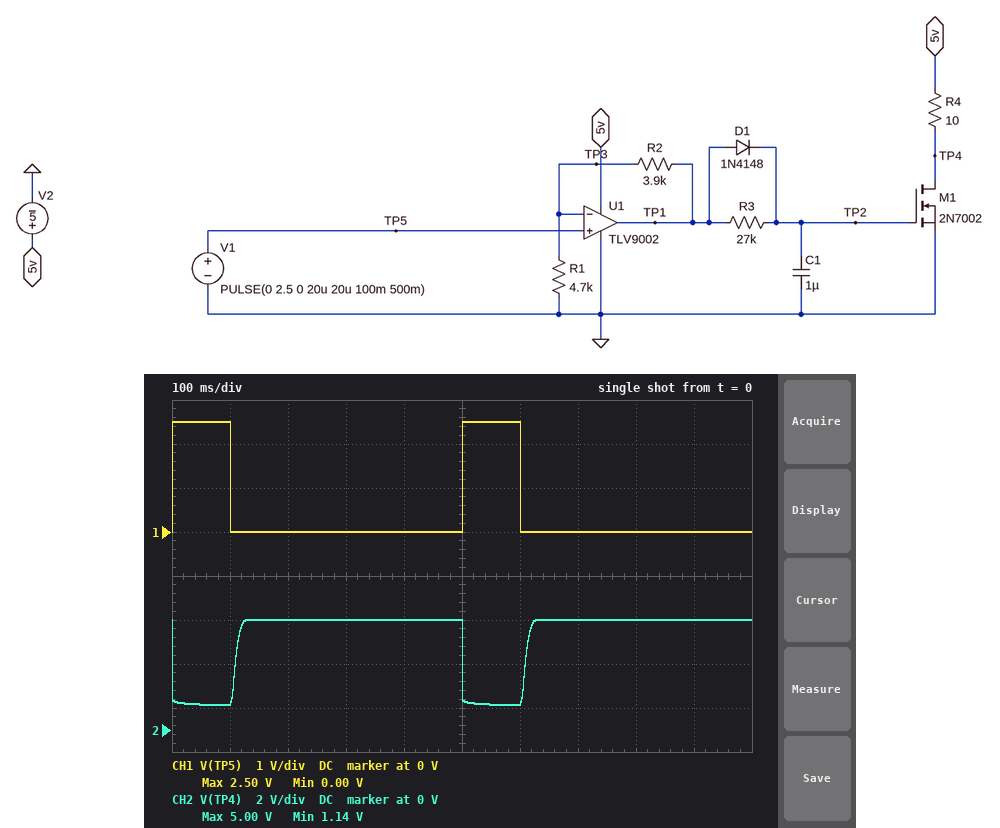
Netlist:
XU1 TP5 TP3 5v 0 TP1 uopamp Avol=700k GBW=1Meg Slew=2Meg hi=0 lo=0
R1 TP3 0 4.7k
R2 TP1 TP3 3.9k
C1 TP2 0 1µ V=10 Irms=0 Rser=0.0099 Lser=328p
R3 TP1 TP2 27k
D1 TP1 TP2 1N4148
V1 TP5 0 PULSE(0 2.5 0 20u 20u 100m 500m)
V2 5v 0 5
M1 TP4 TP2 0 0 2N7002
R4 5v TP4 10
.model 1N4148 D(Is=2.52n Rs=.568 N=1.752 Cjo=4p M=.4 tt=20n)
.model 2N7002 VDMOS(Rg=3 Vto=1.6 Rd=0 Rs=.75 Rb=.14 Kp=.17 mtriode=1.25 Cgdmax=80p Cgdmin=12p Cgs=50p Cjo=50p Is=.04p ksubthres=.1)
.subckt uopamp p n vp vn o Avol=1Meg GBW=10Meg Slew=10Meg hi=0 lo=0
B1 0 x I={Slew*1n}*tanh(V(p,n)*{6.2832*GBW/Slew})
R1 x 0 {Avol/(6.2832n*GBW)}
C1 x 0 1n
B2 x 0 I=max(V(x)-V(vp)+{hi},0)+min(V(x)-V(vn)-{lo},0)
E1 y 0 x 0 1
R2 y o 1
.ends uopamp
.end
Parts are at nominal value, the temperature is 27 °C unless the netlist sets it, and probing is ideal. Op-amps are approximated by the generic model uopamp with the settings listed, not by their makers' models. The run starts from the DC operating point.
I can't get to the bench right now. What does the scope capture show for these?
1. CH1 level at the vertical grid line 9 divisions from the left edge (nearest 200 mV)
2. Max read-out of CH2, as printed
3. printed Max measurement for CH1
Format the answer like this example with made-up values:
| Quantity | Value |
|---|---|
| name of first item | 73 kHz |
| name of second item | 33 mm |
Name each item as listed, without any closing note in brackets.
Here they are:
| Quantity | Value |
|---|---|
| CH1 level at the vertical grid line 9 divisions from the left edge | 0 V |
| Max read-out of CH2, as printed | 5.00 V |
| printed Max measurement for CH1 | 2.50 V |
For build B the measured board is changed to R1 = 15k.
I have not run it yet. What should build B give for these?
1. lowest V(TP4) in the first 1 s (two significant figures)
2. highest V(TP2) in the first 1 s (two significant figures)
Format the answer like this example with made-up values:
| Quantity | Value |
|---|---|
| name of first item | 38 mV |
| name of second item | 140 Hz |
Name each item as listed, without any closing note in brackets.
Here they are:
| Quantity | Value |
|---|---|
| lowest V(TP4) in the first 1 s | 3.3 V |
| highest V(TP2) in the first 1 s | 3.1 V |
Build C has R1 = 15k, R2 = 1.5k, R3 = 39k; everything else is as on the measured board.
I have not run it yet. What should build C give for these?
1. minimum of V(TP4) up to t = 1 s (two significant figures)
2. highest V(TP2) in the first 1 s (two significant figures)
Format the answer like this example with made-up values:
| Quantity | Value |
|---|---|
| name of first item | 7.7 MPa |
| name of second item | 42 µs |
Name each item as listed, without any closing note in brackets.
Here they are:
| Quantity | Value |
|---|---|
| minimum of V(TP4) up to t = 1 s | 4.1 V |
| highest V(TP2) in the first 1 s | 2.7 V |
